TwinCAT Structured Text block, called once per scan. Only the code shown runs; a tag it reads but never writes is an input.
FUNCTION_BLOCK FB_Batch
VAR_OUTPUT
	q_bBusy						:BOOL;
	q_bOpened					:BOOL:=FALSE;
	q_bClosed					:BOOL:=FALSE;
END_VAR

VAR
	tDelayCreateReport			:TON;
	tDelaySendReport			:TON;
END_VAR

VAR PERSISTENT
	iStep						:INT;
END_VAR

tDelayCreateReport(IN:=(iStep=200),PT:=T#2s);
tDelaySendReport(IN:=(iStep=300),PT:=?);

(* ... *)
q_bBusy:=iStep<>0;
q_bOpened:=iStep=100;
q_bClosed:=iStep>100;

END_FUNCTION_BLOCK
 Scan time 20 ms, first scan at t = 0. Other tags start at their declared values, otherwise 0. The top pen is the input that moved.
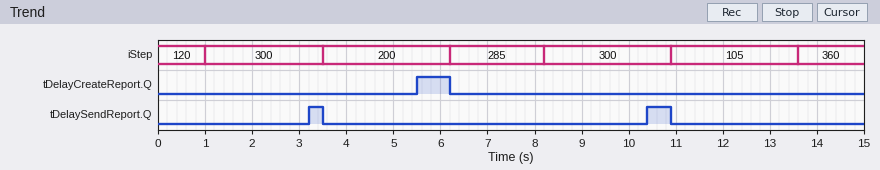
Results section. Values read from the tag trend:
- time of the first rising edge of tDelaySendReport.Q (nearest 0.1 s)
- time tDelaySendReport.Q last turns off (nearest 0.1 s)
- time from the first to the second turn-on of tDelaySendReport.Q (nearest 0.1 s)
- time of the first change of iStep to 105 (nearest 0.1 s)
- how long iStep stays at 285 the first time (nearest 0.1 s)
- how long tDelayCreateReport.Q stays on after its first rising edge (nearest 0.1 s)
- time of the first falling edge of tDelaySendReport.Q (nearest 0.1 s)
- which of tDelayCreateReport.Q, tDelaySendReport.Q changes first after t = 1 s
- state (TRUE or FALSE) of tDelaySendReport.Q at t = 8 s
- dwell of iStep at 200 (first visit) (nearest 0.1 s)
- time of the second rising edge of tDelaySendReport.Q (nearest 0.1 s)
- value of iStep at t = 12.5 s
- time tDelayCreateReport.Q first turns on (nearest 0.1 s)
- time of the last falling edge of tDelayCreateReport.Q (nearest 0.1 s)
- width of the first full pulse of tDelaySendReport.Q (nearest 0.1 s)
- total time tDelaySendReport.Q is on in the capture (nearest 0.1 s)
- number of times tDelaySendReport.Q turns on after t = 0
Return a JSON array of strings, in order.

["3.2 s", "10.9 s", "7.2 s", "10.9 s", "2.0 s", "0.7 s", "3.5 s", "tDelaySendReport.Q", "FALSE", "2.7 s", "10.4 s", "105", "5.5 s", "6.2 s", "0.3 s", "0.8 s", "2"]
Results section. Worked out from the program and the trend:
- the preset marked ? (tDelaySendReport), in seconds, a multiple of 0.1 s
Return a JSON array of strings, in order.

["2.2 s"]
